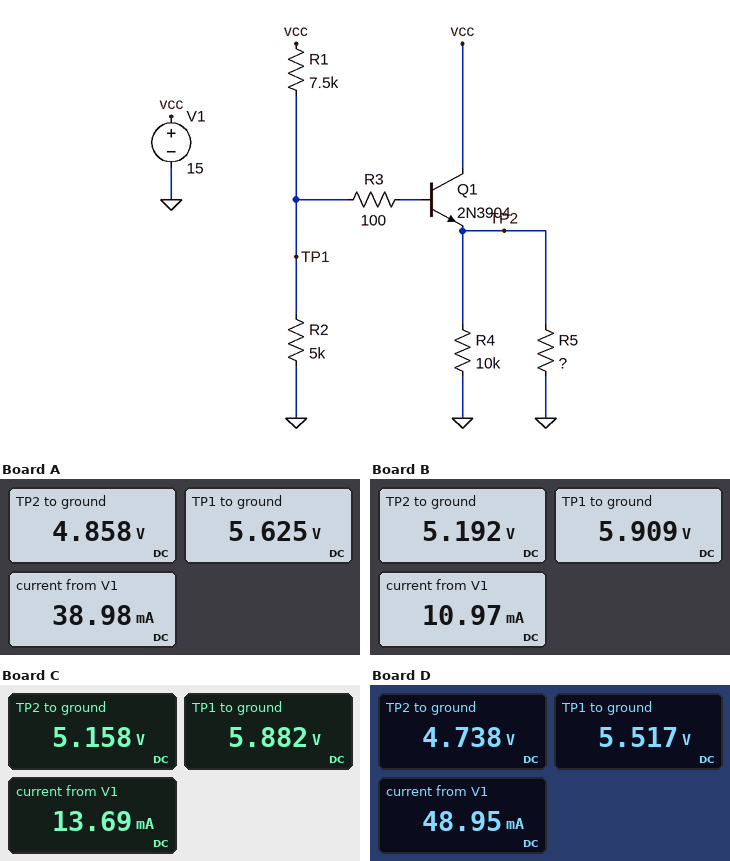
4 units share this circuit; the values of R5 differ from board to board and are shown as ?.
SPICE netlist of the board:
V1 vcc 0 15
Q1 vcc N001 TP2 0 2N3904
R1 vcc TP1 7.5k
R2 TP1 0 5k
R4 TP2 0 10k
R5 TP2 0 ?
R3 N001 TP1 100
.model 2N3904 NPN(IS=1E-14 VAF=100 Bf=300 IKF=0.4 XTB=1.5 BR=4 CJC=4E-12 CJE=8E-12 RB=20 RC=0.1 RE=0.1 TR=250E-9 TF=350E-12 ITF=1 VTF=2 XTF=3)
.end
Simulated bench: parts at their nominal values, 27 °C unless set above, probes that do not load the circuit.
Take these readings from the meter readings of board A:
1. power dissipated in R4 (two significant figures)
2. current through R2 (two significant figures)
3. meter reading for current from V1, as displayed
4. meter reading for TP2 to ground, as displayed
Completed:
2.4 mW
1.1 mA
38.98 mA
4.858 V
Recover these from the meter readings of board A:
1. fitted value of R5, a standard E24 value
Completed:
130 Ω
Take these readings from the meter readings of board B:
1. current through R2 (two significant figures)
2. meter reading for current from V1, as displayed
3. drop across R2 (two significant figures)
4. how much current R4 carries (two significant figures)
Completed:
1.2 mA
10.97 mA
5.9 V
520 µA
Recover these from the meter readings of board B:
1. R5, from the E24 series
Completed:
560 Ω
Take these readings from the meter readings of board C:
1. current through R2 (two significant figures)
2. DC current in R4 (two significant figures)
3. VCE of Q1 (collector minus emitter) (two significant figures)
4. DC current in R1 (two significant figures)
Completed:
1.2 mA
520 µA
9.8 V
1.2 mA
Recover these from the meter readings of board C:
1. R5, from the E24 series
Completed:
430 Ω
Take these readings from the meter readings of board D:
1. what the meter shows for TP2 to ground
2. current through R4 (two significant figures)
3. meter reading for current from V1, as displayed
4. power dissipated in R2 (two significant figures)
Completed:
4.738 V
470 µA
48.95 mA
6.1 mW
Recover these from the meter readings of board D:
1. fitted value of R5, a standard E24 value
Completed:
100 Ω
